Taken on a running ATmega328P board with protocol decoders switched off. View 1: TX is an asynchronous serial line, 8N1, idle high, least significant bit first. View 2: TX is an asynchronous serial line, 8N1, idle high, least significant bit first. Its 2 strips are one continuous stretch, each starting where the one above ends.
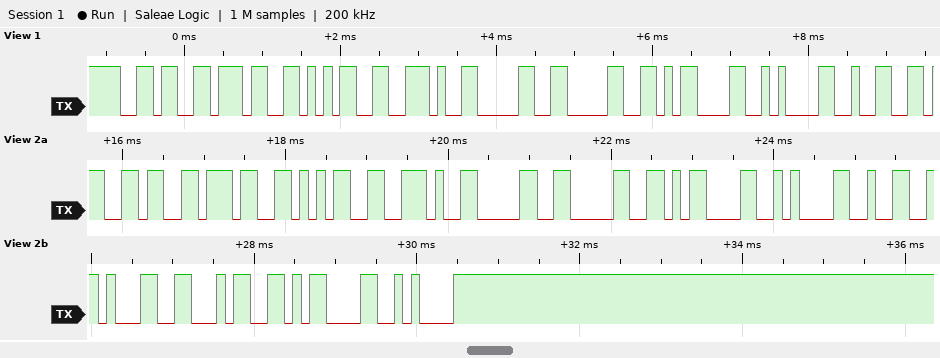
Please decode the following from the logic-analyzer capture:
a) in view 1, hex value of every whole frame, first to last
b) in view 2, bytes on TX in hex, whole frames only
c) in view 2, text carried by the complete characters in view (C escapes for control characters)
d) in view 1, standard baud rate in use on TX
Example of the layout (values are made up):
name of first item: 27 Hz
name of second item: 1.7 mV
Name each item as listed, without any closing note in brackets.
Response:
in view 1, hex value of every whole frame, first to last: 36 37 35 2E 30 30 0D 0A 32
in view 2, bytes on TX in hex, whole frames only: 36 37 35 2E 30 30 0D 0A 32 31 34 0D 0A
in view 2, text carried by the complete characters in view: "675.00\r\n214\r\n"
in view 1, standard baud rate in use on TX: 9600 baud
